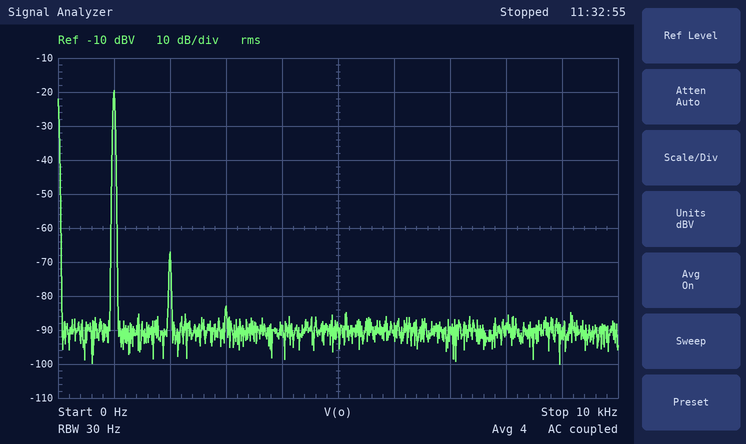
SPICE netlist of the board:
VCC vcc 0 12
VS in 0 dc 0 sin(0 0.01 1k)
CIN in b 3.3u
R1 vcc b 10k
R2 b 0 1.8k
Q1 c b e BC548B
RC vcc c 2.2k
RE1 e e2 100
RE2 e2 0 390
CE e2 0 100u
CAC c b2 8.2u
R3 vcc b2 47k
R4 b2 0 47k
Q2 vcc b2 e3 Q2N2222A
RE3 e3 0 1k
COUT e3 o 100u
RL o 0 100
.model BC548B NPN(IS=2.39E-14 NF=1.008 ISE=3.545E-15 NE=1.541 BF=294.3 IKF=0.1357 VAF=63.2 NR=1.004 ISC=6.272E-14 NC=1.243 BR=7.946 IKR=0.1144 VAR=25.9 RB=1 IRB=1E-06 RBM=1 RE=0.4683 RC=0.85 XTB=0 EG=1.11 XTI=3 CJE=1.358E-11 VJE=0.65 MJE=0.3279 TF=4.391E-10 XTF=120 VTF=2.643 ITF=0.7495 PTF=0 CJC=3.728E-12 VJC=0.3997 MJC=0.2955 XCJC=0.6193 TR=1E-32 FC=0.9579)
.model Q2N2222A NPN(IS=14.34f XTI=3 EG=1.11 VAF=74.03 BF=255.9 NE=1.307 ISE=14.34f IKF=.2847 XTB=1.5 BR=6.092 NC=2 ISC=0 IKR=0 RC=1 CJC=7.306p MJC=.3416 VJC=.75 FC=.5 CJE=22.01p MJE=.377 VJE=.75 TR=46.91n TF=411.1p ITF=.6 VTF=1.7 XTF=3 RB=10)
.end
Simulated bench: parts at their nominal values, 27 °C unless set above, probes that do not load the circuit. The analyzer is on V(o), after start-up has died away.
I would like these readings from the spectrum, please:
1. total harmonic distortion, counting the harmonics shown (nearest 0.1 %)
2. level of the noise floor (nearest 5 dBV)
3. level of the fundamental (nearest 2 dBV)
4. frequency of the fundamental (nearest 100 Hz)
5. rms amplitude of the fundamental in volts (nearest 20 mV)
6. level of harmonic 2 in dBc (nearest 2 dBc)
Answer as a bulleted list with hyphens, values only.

- 0.4 %
- -90 dBV
- -20 dBV
- 1.0 kHz
- 100 mV
- -48 dBc
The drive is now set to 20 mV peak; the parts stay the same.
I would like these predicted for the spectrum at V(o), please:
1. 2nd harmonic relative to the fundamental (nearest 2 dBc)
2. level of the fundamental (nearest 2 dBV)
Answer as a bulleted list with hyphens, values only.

- -40 dBc
- -14 dBV
